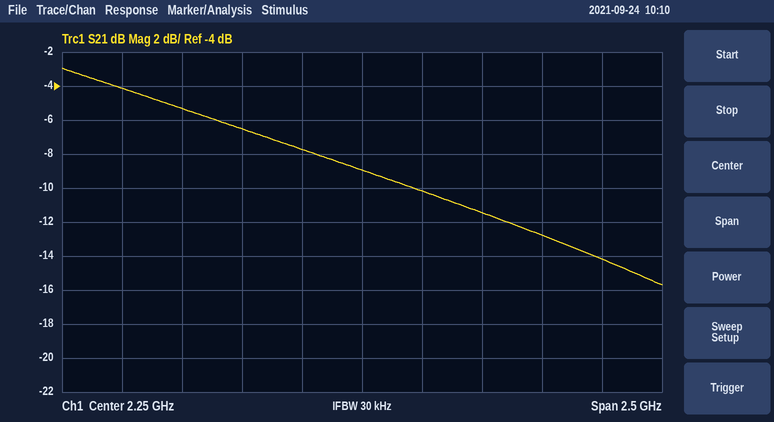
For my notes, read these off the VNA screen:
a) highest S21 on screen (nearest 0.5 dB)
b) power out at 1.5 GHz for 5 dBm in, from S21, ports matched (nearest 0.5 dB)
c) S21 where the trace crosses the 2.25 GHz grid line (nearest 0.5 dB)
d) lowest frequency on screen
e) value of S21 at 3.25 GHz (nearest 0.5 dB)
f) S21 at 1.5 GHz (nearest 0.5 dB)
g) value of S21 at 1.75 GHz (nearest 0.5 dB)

-3.0 dB
-0.5 dBm
-9.0 dB
1 GHz
-14.0 dB
-5.5 dB
-6.5 dB
